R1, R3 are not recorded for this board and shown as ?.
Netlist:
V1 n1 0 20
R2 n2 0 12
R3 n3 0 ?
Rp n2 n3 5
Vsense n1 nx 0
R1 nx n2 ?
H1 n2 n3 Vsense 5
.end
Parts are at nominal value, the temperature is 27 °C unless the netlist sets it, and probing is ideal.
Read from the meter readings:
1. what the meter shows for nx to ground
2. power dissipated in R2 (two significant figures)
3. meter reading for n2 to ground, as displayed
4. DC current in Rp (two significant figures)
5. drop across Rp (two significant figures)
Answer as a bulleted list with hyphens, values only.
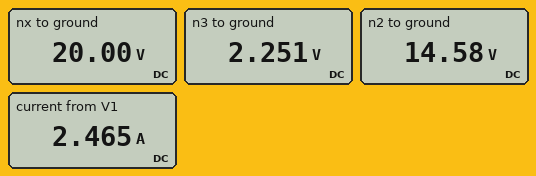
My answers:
- 20.00 V
- 18 W
- 14.58 V
- 2.5 A
- 12 V
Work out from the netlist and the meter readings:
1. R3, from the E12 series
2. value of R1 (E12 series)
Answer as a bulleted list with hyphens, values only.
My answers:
- 1.8 Ω
- 2.2 Ω
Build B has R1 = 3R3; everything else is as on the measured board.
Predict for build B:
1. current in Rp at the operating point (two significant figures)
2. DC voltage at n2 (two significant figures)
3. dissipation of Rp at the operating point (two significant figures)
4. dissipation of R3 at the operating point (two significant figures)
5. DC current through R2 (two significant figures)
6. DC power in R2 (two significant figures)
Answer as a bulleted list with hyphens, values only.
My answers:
- 2.2 A
- 13 V
- 24 W
- 2.2 W
- 1.1 A
- 14 W
